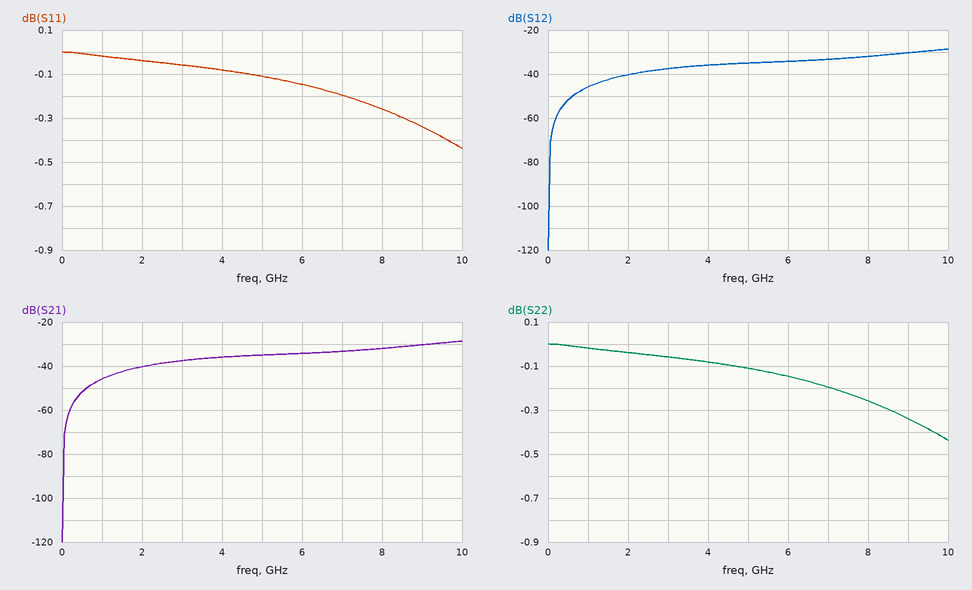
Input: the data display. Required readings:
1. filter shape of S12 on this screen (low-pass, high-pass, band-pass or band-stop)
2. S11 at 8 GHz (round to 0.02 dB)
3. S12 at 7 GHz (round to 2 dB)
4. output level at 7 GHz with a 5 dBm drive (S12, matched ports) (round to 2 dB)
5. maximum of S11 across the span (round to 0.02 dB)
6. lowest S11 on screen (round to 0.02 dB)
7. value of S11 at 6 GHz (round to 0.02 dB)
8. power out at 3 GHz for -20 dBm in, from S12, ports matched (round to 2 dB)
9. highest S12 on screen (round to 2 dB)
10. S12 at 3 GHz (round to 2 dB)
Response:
high-pass
-0.26 dB
-34 dB
-28 dBm
0.00 dB
-0.44 dB
-0.14 dB
-58 dBm
-28 dB
-38 dB
